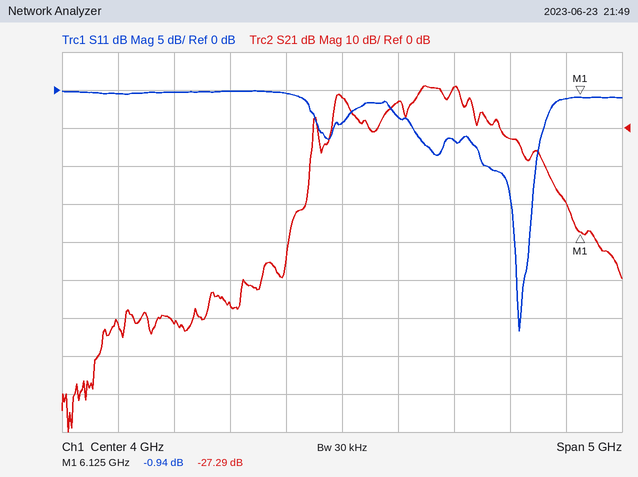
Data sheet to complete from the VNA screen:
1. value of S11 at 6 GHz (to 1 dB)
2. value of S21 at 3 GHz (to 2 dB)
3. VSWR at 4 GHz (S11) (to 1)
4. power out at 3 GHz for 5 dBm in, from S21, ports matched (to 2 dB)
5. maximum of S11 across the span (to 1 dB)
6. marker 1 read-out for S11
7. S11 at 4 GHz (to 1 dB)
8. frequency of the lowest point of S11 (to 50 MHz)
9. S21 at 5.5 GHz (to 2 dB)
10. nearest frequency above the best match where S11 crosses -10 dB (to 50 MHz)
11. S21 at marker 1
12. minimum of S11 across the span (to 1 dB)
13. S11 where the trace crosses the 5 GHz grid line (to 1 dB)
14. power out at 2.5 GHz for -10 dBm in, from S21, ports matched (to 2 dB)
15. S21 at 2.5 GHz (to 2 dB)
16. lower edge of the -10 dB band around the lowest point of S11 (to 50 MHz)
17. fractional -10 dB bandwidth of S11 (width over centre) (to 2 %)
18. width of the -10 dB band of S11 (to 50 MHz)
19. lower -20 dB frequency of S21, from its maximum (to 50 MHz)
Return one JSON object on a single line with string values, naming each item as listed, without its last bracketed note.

{"value of S11 at 6 GHz": "-1 dB", "value of S21 at 3 GHz": "-46 dB", "VSWR at 4 GHz (S11)": "4", "power out at 3 GHz for 5 dBm in, from S21, ports matched": "-42 dBm", "maximum of S11 across the span": "0 dB", "marker 1 read-out for S11": "-0.94 dB", "S11 at 4 GHz": "-4 dB", "frequency of the lowest point of S11": "5.60 GHz", "S21 at 5.5 GHz": "-2 dB", "nearest frequency above the best match where S11 crosses -10 dB": "5.75 GHz", "S21 at marker 1": "-27.29 dB", "minimum of S11 across the span": "-32 dB", "S11 where the trace crosses the 5 GHz grid line": "-7 dB", "power out at 2.5 GHz for -10 dBm in, from S21, ports matched": "-62 dBm", "S21 at 2.5 GHz": "-52 dB", "lower edge of the -10 dB band around the lowest point of S11": "5.30 GHz", "fractional -10 dB bandwidth of S11 (width over centre)": "8 %", "width of the -10 dB band of S11": "450 MHz", "lower -20 dB frequency of S21, from its maximum": "3.70 GHz"}
